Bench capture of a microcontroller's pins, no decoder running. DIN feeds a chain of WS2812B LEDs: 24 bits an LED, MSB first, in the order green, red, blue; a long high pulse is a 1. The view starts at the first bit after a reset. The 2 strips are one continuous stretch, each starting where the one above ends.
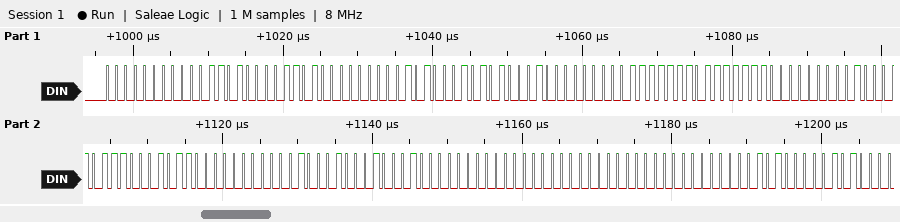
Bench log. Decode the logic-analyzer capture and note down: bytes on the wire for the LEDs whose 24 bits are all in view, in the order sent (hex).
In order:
00 1A 1A 00 A2 A2 00 FE FE 00 8B 8B 00 11 11 00 00 00 00 0A 0A
